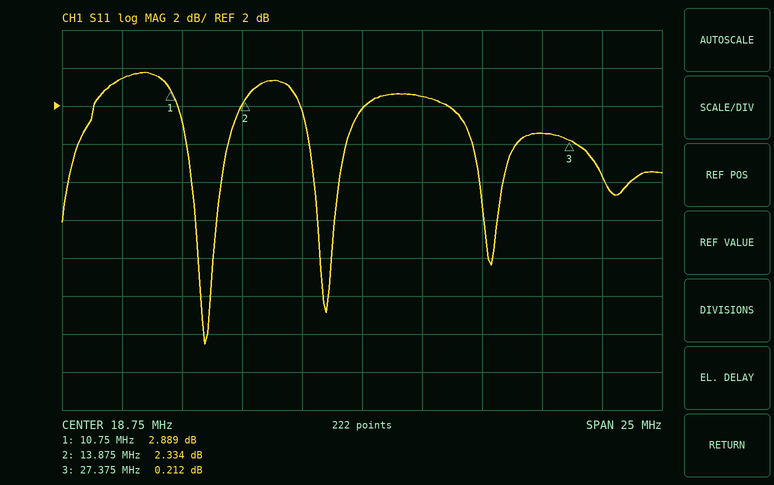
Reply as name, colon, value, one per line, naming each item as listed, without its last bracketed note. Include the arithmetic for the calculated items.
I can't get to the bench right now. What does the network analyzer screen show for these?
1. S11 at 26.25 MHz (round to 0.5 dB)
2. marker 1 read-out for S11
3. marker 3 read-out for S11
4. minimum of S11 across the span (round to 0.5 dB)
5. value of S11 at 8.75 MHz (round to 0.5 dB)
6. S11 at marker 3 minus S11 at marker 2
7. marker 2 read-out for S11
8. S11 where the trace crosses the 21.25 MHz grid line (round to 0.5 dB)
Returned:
S11 at 26.25 MHz: 0.5 dB
marker 1 read-out for S11: 2.889 dB
marker 3 read-out for S11: 0.212 dB
minimum of S11 across the span: -10.5 dB
value of S11 at 8.75 MHz: 3.5 dB
S11 at marker 3 minus S11 at marker 2: 0.212 − (2.334) = -2.122 dB
marker 2 read-out for S11: 2.334 dB
S11 where the trace crosses the 21.25 MHz grid line: 2.5 dB
